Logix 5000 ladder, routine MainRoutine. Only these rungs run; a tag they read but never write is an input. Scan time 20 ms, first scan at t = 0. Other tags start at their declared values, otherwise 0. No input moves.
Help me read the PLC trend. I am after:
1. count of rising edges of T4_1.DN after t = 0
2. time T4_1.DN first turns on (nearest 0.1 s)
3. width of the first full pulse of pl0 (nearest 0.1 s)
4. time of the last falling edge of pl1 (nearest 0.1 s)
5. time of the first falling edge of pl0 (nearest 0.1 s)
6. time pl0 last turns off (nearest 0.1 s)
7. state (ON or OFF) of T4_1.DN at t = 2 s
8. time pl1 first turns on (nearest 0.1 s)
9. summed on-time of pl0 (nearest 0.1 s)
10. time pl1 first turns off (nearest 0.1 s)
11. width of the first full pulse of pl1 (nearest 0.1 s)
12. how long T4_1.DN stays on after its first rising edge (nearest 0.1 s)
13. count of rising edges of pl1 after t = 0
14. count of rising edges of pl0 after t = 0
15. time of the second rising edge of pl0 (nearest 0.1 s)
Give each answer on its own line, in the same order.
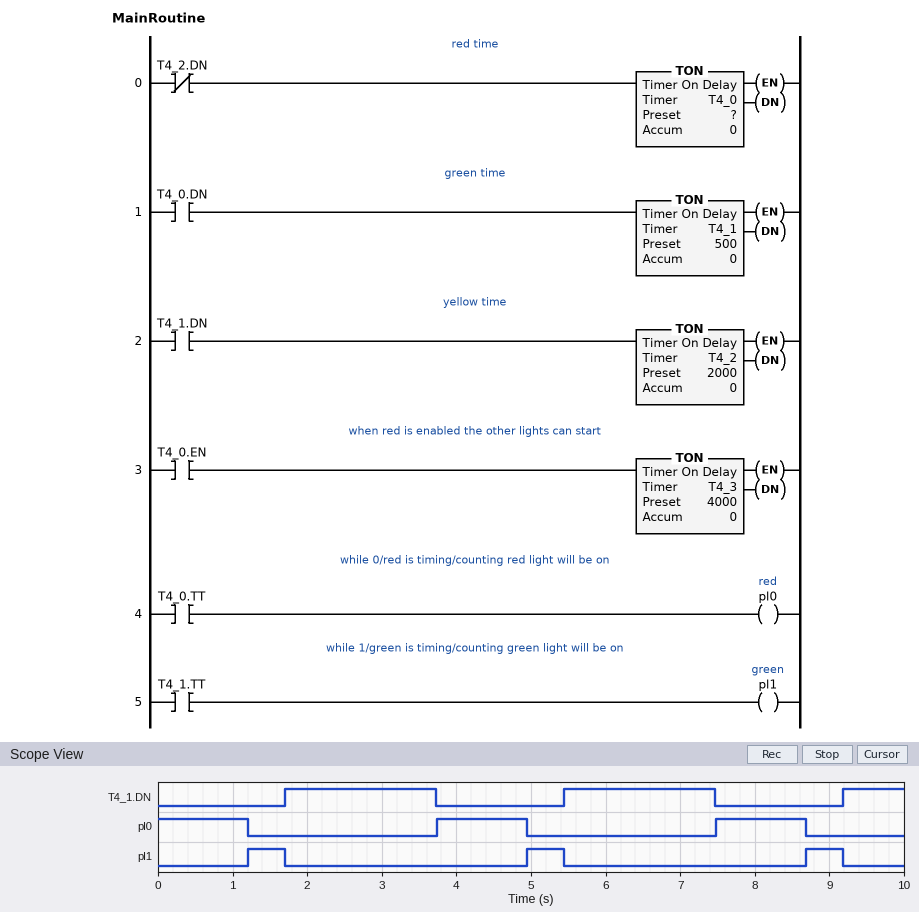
3
1.7 s
1.2 s
9.2 s
1.2 s
8.7 s
ON
1.2 s
3.6 s
1.7 s
0.5 s
2.0 s
3
2
7.5 s
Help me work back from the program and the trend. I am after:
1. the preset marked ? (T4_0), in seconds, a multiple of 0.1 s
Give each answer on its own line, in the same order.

1.2 s
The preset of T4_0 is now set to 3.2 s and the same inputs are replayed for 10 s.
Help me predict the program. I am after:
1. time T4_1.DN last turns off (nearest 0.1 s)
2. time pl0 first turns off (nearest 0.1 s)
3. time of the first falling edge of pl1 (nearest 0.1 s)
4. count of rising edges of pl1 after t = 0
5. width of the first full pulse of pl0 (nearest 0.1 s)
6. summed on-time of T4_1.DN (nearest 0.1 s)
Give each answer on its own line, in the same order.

5.7 s
3.2 s
3.7 s
2
3.2 s
2.6 s
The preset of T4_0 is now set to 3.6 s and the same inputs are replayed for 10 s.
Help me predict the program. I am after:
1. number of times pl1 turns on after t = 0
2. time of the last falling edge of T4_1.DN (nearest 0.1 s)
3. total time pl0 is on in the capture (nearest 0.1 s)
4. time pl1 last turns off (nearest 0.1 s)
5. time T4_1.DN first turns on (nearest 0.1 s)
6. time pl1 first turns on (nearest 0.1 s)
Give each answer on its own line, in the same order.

2
6.1 s
7.2 s
4.1 s
4.1 s
3.6 s
